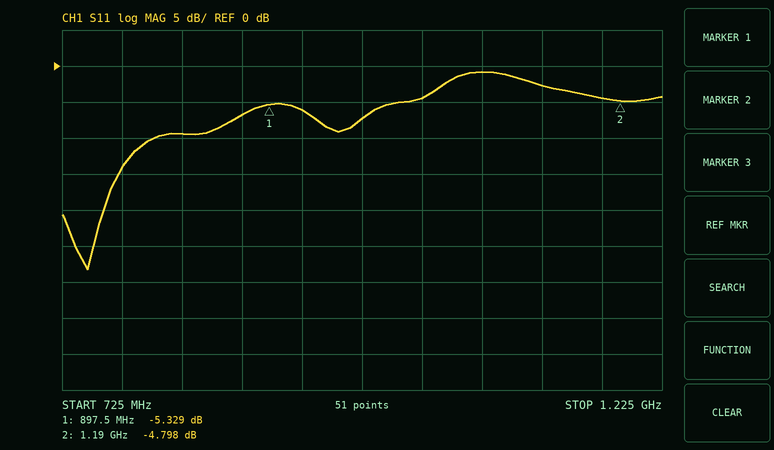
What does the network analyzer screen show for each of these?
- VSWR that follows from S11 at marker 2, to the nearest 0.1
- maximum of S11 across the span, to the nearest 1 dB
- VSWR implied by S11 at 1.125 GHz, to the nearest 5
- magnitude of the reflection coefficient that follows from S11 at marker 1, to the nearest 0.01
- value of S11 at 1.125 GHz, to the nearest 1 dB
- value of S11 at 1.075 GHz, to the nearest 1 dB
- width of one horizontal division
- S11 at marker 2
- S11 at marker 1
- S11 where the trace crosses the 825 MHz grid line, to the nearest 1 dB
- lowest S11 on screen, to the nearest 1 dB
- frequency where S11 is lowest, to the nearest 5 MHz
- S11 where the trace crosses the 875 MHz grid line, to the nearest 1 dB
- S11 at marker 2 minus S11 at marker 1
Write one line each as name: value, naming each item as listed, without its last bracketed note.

VSWR that follows from S11 at marker 2, to the nearest 0.1: 3.7
maximum of S11 across the span, to the nearest 1 dB: -1 dB
VSWR implied by S11 at 1.125 GHz, to the nearest 5: 5
magnitude of the reflection coefficient that follows from S11 at marker 1, to the nearest 0.01: 0.54
value of S11 at 1.125 GHz, to the nearest 1 dB: -3 dB
value of S11 at 1.075 GHz, to the nearest 1 dB: -1 dB
width of one horizontal division: 50 MHz
S11 at marker 2: -4.798 dB
S11 at marker 1: -5.329 dB
S11 where the trace crosses the 825 MHz grid line, to the nearest 1 dB: -9 dB
lowest S11 on screen, to the nearest 1 dB: -28 dB
frequency where S11 is lowest, to the nearest 5 MHz: 745 MHz
S11 where the trace crosses the 875 MHz grid line, to the nearest 1 dB: -7 dB
S11 at marker 2 minus S11 at marker 1: 0.531 dB
